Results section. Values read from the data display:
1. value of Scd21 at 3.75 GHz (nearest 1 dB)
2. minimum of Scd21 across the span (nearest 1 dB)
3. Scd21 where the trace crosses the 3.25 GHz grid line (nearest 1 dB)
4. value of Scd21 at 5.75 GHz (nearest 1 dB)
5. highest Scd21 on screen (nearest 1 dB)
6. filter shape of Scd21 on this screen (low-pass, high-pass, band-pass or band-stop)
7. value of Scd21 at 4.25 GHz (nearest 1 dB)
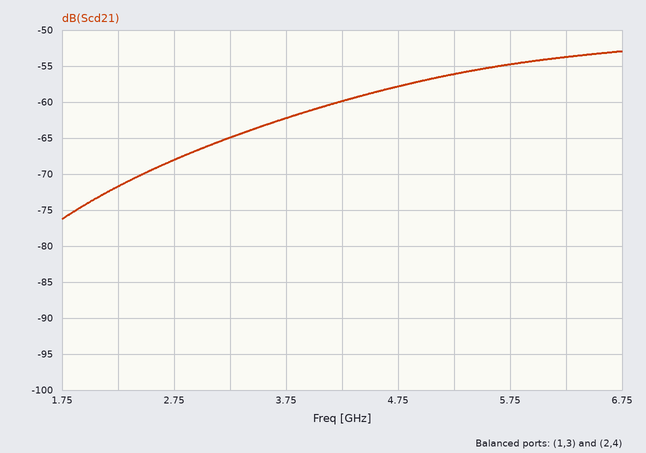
-62 dB
-76 dB
-65 dB
-55 dB
-53 dB
high-pass
-60 dB
